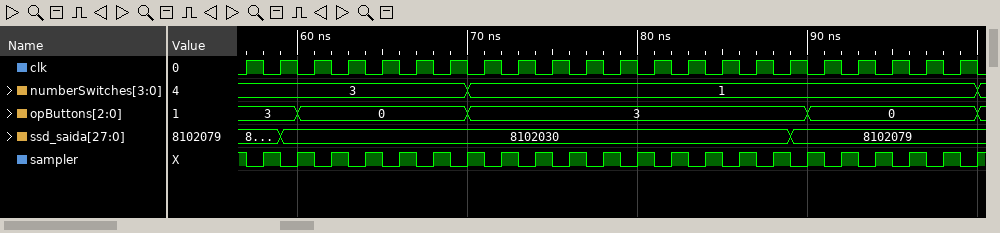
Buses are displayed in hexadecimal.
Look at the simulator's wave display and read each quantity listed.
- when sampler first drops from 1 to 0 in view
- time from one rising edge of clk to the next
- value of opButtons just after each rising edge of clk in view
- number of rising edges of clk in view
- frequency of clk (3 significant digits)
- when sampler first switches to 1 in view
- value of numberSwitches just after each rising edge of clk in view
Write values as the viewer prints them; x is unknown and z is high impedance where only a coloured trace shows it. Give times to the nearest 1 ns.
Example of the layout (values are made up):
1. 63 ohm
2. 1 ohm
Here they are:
1. 57 ns
2. 2 ns
3. 3, 3, 0, 0, 0, 0, 0, 3, 3, 3, 3, 3, 3, 3, 3, 3, 3, 0, 0, 0, 0, 0
4. 22
5. 500 MHz
6. 58 ns
7. 3, 3, 3, 3, 3, 3, 3, 1, 1, 1, 1, 1, 1, 1, 1, 1, 1, 1, 1, 1, 1, 1
